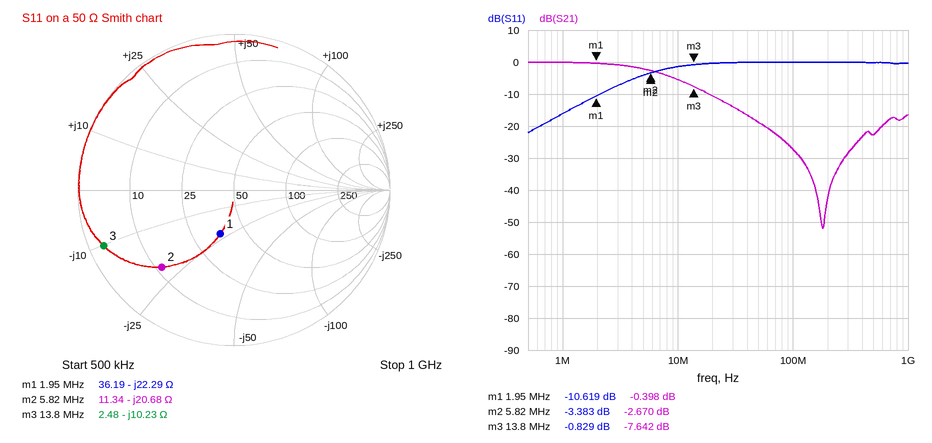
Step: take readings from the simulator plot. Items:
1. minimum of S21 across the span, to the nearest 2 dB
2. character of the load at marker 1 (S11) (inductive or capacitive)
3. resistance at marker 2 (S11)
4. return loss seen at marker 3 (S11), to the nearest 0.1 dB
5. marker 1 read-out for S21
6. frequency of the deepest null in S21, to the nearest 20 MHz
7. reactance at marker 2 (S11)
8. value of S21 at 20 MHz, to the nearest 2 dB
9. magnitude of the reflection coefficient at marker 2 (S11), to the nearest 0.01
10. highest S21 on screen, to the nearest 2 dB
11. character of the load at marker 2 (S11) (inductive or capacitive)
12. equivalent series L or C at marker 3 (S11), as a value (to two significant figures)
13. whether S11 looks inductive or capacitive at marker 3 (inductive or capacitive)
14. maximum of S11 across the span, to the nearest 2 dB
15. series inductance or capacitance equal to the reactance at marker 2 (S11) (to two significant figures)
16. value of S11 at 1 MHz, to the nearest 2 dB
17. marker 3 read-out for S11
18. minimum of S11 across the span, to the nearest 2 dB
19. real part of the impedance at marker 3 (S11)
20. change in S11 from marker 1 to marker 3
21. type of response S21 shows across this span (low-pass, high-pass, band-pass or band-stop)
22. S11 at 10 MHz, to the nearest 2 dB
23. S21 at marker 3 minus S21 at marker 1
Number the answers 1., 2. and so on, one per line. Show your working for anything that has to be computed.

1. -52 dB
2. capacitive
3. 11.34 Ω
4. 0.8 dB
5. -0.398 dB
6. 180 MHz
7. -20.68 Ω
8. -10 dB
9. 0.68
10. 0 dB
11. capacitive
12. C = 1/(2π × 13.8 MHz × 10.23 Ω) ≈ 1.1 nF
13. capacitive
14. 0 dB
15. C = 1/(2π × 5.82 MHz × 20.68 Ω) ≈ 1.3 nF
16. -16 dB
17. -0.829 dB
18. -22 dB
19. 2.48 Ω
20. -0.829 − (-10.619) = 9.790 dB
21. low-pass
22. -2 dB
23. -7.642 − (-0.398) = -7.244 dB
